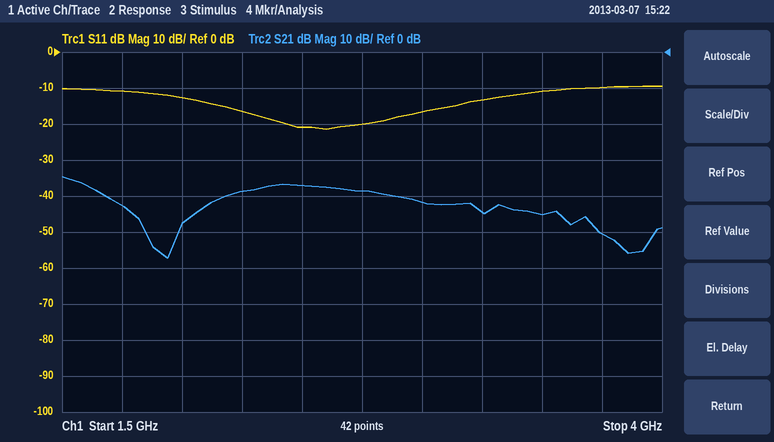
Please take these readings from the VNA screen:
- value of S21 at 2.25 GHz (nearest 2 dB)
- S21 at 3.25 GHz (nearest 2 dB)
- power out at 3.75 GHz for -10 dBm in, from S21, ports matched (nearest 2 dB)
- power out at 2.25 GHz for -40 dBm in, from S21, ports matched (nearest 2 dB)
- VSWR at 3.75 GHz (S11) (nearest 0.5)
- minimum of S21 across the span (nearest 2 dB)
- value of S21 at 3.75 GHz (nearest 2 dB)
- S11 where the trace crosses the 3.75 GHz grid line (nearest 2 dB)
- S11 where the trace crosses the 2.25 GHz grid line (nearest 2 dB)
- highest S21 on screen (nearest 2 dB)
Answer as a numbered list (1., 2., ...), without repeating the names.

1. -38 dB
2. -44 dB
3. -60 dBm
4. -78 dBm
5. 2.0
6. -58 dB
7. -50 dB
8. -10 dB
9. -16 dB
10. -34 dB
